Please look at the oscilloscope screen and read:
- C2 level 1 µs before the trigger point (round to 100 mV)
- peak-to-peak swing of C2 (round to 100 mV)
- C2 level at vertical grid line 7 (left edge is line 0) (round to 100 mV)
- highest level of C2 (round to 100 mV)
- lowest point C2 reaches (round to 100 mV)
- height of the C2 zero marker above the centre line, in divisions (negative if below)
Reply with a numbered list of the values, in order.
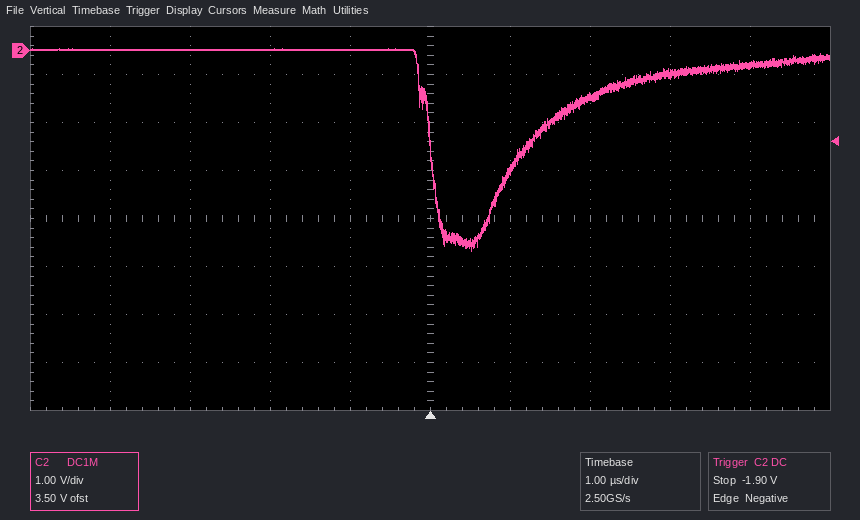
1. 0.0 V
2. 4.2 V
3. -1.0 V
4. 0.0 V
5. -4.2 V
6. +3.5 div
